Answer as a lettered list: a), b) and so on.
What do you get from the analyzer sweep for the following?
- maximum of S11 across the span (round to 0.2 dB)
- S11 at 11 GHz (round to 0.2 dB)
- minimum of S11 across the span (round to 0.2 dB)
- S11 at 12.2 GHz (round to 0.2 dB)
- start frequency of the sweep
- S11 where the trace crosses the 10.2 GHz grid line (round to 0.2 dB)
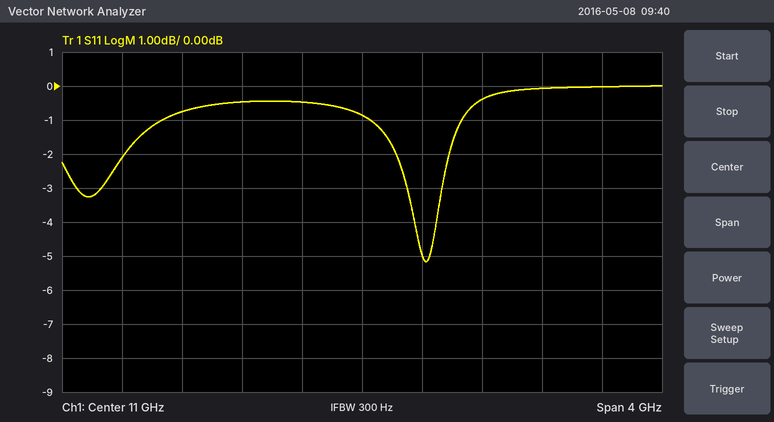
a) 0.0 dB
b) -0.8 dB
c) -5.2 dB
d) 0.0 dB
e) 9 GHz
f) -0.4 dB
